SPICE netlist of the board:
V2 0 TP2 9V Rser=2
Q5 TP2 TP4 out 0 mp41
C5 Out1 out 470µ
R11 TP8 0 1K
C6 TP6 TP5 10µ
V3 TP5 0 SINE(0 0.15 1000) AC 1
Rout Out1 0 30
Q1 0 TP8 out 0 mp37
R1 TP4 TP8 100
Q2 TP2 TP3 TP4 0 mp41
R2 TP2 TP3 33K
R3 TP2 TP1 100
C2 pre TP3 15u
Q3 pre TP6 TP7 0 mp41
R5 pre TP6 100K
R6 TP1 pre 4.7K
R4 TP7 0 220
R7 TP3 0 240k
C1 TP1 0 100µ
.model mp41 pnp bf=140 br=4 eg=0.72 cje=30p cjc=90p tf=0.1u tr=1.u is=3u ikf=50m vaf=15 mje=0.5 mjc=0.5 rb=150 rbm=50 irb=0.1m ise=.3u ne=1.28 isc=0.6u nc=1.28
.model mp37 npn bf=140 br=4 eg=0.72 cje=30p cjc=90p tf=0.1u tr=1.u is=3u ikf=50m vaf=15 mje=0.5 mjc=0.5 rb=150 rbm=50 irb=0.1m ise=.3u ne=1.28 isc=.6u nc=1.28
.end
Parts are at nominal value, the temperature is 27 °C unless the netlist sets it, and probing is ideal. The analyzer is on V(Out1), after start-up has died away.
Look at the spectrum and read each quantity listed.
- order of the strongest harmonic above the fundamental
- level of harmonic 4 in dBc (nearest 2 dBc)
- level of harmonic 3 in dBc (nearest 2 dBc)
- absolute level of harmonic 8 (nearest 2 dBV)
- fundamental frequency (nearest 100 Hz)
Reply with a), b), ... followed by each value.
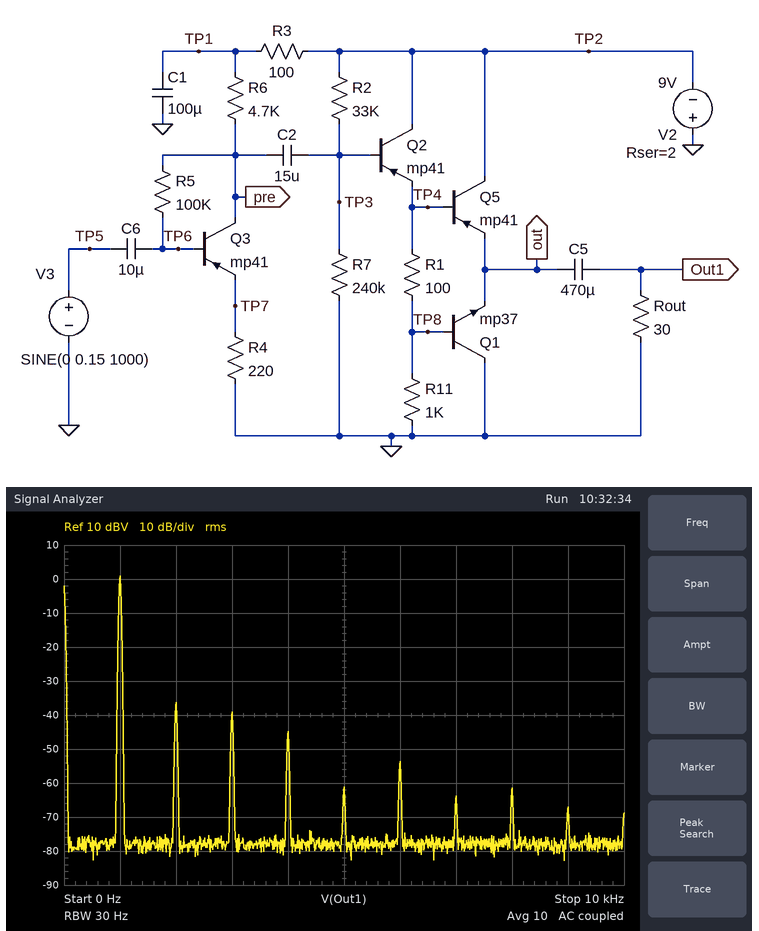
a) 2
b) -46 dBc
c) -40 dBc
d) -62 dBV
e) 1.0 kHz
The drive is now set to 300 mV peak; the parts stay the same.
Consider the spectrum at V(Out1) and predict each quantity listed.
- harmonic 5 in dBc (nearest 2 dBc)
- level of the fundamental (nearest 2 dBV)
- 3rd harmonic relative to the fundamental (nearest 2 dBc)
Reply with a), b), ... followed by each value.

a) -40 dBc
b) 6 dBV
c) -20 dBc
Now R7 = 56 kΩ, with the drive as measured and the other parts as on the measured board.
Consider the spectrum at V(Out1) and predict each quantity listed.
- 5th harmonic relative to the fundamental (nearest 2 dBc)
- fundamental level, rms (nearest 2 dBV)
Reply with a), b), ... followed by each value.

a) -50 dBc
b) 0 dBV
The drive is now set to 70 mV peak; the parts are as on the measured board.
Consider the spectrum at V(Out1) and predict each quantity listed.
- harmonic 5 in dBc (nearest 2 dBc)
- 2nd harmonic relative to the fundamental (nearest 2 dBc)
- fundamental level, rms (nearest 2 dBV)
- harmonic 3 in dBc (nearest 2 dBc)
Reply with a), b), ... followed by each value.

a) -58 dBc
b) -34 dBc
c) -6 dBV
d) -46 dBc
